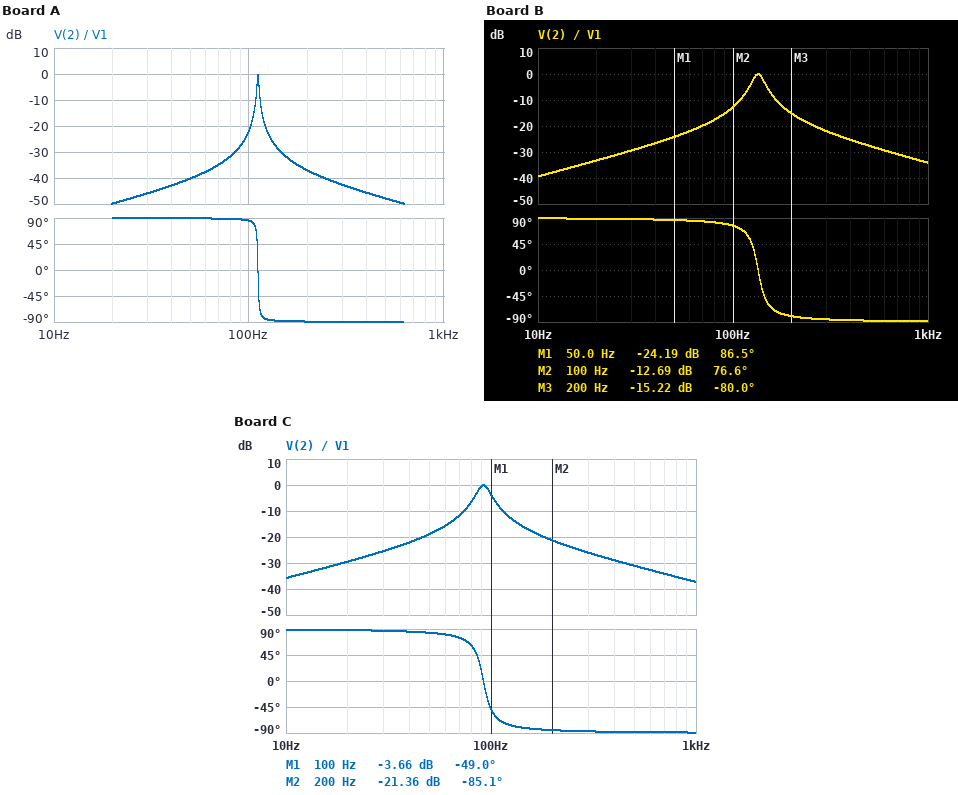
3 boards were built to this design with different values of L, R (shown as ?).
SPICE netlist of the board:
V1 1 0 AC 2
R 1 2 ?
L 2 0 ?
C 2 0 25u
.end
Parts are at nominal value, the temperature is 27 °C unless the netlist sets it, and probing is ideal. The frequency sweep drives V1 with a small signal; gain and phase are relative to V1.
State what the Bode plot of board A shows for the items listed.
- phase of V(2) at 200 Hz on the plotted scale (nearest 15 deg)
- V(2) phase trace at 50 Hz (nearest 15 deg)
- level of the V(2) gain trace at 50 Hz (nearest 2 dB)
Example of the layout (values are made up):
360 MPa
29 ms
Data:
-90 deg
90 deg
-40 dB
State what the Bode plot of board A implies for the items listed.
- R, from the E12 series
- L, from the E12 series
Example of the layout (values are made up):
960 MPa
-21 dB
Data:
3.3 kΩ
82 mH
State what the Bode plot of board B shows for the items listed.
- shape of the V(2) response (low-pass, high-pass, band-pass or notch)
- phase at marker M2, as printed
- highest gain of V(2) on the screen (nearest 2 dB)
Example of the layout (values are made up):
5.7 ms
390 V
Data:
band-pass
76.6 deg
0 dB
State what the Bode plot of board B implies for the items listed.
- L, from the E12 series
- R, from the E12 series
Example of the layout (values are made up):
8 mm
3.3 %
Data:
56 mH
330 Ω
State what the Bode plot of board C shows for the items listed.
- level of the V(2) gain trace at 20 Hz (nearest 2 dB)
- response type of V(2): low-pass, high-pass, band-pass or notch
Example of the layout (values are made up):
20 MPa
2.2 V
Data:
-30 dB
band-pass
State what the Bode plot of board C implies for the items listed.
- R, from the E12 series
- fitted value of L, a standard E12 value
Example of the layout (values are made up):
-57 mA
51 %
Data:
470 Ω
120 mH
